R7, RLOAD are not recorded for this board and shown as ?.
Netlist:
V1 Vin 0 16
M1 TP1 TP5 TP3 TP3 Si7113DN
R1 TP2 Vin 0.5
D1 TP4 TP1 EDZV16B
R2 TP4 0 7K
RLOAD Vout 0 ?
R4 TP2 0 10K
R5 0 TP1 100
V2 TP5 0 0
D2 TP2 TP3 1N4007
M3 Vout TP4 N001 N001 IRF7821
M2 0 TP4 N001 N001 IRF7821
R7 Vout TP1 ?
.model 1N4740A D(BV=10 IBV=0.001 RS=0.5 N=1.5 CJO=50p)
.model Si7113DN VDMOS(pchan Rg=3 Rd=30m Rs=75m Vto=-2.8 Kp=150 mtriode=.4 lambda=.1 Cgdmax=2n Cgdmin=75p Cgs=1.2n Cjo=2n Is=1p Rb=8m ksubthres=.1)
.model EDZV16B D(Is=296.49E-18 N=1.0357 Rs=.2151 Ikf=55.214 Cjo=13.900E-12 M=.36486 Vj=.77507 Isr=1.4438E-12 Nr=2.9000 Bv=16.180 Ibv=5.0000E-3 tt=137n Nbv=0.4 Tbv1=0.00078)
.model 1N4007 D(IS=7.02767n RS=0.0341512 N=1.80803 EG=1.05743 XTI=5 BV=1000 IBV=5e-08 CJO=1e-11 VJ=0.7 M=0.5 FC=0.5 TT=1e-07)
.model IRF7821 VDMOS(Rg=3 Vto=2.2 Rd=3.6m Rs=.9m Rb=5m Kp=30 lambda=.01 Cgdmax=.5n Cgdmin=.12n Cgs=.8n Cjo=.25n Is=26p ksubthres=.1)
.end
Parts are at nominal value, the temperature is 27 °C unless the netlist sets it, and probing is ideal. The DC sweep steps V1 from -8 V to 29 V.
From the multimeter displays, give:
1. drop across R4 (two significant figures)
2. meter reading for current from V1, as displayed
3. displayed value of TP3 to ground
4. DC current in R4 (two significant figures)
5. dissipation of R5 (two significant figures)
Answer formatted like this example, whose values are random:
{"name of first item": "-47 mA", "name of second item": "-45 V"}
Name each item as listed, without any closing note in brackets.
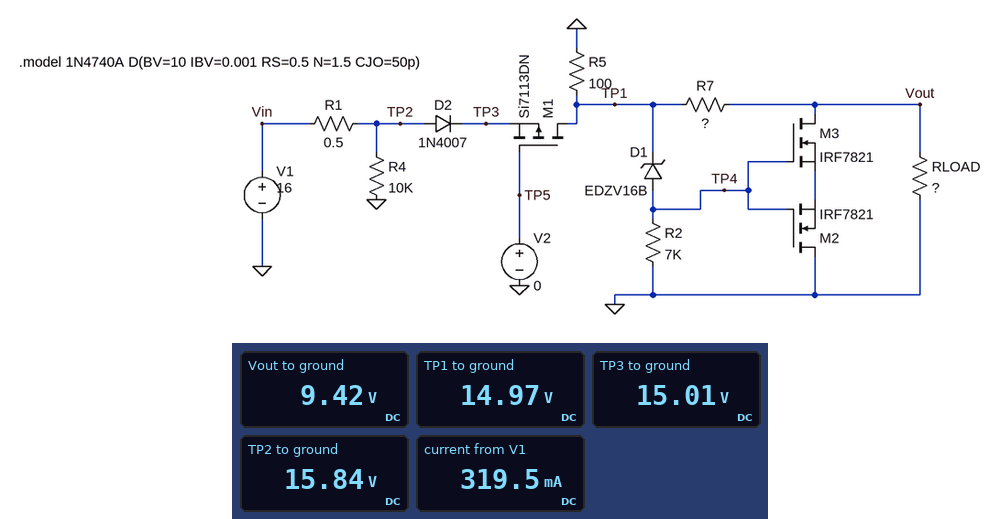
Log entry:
{"drop across R4": "16 V", "meter reading for current from V1, as displayed": "319.5 mA", "displayed value of TP3 to ground": "15.01 V", "DC current in R4": "1.6 mA", "dissipation of R5": "2.2 W"}
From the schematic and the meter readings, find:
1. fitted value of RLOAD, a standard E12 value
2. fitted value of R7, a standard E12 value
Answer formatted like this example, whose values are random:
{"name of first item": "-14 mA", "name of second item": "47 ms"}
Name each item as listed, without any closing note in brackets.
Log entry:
{"fitted value of RLOAD, a standard E12 value": "56 Ω", "fitted value of R7, a standard E12 value": "33 Ω"}
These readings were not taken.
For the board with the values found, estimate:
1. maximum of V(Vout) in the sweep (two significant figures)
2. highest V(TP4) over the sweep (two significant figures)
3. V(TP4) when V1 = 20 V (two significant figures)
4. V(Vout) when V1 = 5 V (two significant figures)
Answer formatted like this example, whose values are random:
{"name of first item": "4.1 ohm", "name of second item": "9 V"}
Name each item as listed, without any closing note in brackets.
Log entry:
{"maximum of V(Vout) in the sweep": "11 V", "highest V(TP4) over the sweep": "11 V", "V(TP4) when V1 = 20 V": "2.5 V", "V(Vout) when V1 = 5 V": "2.6 V"}
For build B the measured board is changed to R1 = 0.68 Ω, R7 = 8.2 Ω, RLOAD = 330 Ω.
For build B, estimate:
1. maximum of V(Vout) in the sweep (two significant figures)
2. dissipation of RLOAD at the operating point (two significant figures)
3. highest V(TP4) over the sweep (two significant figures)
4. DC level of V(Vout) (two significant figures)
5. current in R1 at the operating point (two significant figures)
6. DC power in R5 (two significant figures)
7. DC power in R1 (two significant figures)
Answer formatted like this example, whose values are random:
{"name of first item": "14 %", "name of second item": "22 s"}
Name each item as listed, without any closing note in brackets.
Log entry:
{"maximum of V(Vout) in the sweep": "18 V", "dissipation of RLOAD at the operating point": "650 mW", "highest V(TP4) over the sweep": "9.2 V", "DC level of V(Vout)": "15 V", "current in R1 at the operating point": "200 mA", "DC power in R5": "2.3 W", "DC power in R1": "26 mW"}
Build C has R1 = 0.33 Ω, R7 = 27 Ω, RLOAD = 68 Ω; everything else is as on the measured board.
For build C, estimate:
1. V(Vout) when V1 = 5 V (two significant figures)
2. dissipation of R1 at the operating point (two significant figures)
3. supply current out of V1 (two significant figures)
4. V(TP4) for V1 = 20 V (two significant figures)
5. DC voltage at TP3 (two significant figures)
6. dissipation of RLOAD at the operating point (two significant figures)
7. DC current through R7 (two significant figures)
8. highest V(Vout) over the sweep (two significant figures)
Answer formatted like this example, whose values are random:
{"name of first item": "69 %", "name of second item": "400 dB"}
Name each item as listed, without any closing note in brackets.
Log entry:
{"V(Vout) when V1 = 5 V": "3.0 V", "dissipation of R1 at the operating point": "32 mW", "supply current out of V1": "310 mA", "V(TP4) for V1 = 20 V": "2.6 V", "DC voltage at TP3": "15 V", "dissipation of RLOAD at the operating point": "1.7 W", "DC current through R7": "160 mA", "highest V(Vout) over the sweep": "13 V"}
